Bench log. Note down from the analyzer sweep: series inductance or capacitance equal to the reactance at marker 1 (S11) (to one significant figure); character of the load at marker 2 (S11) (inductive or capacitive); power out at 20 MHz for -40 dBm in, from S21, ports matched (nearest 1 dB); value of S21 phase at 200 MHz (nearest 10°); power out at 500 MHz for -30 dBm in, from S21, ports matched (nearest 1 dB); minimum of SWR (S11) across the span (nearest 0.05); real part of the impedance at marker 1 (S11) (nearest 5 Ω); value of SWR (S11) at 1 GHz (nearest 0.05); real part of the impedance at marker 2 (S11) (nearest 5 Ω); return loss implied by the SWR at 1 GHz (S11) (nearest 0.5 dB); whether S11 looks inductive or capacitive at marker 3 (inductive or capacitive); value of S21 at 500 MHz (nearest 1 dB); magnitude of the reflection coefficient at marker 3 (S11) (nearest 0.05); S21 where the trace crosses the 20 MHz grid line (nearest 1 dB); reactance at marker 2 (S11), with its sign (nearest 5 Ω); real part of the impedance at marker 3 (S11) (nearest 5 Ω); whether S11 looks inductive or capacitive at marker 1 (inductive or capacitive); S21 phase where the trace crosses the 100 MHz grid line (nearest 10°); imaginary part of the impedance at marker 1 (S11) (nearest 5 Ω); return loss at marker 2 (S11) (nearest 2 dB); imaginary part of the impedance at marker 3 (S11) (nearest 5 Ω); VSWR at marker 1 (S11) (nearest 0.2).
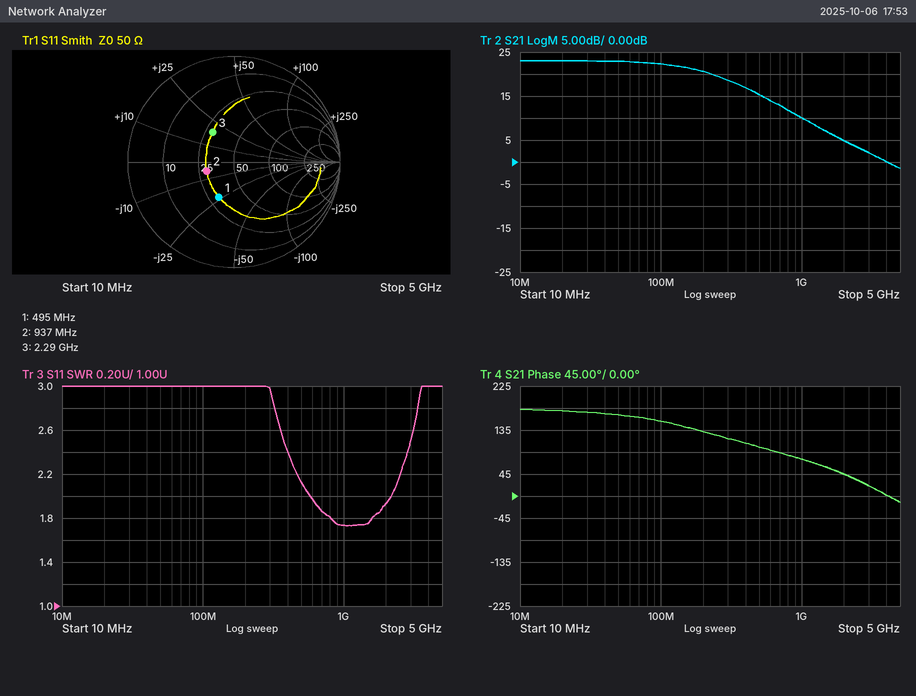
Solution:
10 pF
capacitive
-17 dBm
130°
-15 dBm
1.75
30 Ω
1.75
30 Ω
11.5 dB
inductive
15 dB
0.35
23 dB
-5 Ω
30 Ω
capacitive
150°
-25 Ω
12 dB
+20 Ω
2.2
